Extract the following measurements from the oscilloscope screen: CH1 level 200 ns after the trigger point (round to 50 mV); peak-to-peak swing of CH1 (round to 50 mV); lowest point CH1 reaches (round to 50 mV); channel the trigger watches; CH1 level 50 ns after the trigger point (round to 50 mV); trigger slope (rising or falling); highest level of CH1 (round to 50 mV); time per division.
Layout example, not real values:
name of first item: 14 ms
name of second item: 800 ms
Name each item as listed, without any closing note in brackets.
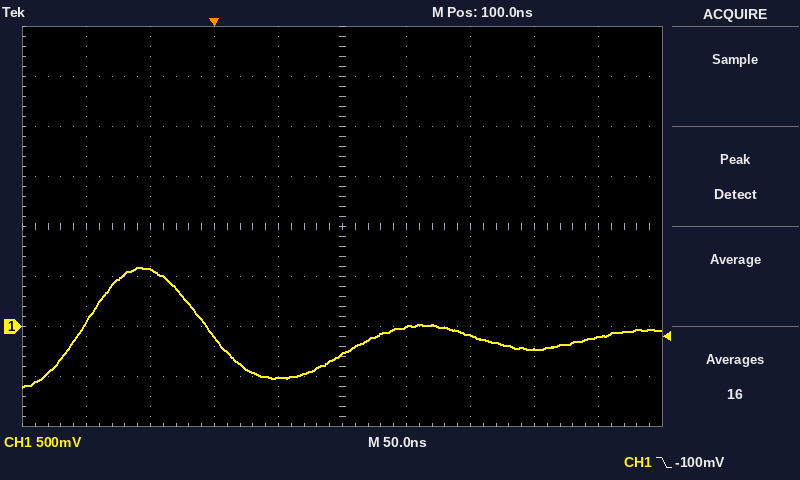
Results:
CH1 level 200 ns after the trigger point: -100 mV
peak-to-peak swing of CH1: 1.20 V
lowest point CH1 reaches: -600 mV
channel the trigger watches: CH1
CH1 level 50 ns after the trigger point: -500 mV
trigger slope: falling
highest level of CH1: 600 mV
time per division: 50 ns
